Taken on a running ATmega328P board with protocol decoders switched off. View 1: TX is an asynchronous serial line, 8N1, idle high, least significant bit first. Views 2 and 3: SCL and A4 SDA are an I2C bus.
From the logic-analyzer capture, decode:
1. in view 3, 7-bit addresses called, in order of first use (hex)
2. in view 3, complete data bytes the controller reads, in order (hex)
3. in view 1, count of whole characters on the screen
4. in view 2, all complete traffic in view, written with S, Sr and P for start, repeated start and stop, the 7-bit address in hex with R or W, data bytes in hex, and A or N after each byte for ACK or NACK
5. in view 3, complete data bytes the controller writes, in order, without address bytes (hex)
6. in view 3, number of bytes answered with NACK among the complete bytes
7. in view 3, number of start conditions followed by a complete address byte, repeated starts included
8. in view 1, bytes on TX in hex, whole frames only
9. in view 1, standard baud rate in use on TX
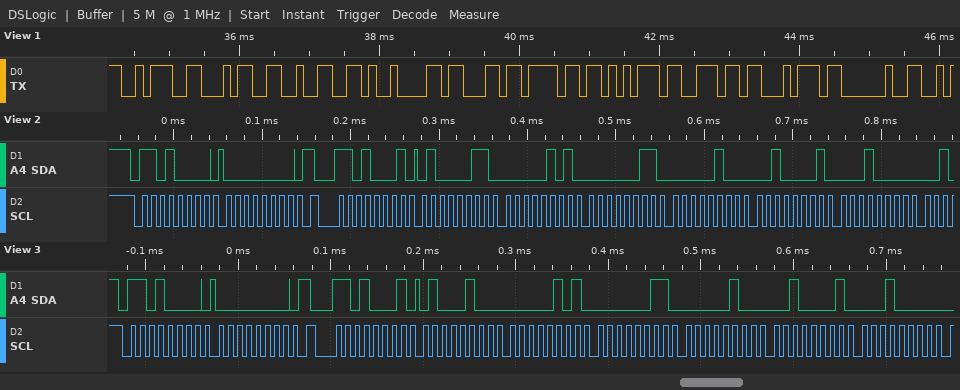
0x68
44 05 03 04 21 10
10
S 68W A 00 A Sr 68R A 43 A 05 A 03 A 04 A 21 A 10 A
00
0
2
3A 34 32 09 63 6F 75 6E 74 20
9600 baud
